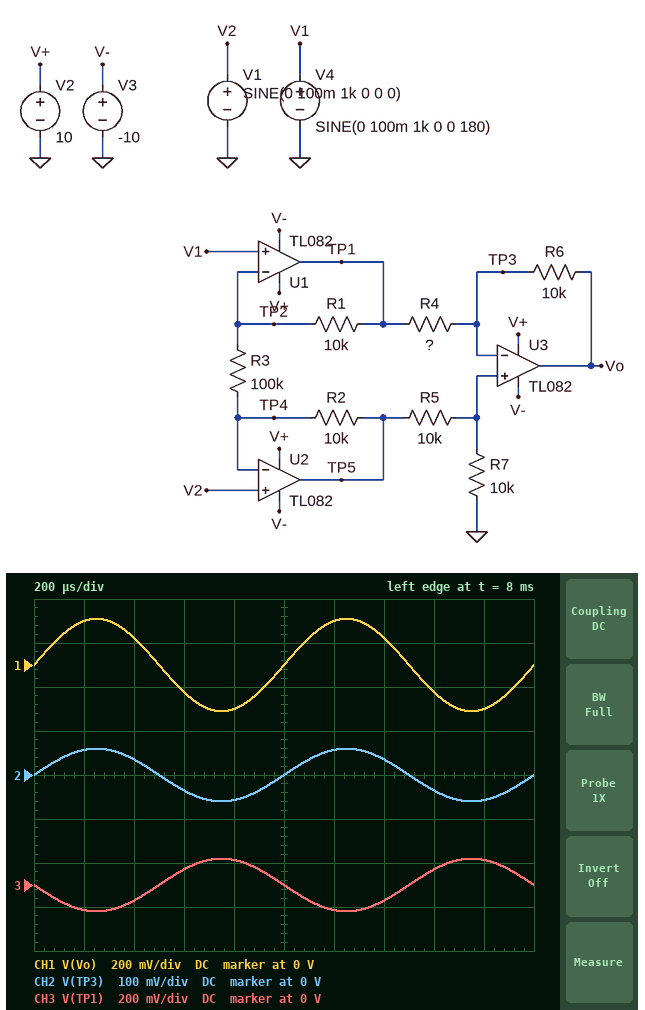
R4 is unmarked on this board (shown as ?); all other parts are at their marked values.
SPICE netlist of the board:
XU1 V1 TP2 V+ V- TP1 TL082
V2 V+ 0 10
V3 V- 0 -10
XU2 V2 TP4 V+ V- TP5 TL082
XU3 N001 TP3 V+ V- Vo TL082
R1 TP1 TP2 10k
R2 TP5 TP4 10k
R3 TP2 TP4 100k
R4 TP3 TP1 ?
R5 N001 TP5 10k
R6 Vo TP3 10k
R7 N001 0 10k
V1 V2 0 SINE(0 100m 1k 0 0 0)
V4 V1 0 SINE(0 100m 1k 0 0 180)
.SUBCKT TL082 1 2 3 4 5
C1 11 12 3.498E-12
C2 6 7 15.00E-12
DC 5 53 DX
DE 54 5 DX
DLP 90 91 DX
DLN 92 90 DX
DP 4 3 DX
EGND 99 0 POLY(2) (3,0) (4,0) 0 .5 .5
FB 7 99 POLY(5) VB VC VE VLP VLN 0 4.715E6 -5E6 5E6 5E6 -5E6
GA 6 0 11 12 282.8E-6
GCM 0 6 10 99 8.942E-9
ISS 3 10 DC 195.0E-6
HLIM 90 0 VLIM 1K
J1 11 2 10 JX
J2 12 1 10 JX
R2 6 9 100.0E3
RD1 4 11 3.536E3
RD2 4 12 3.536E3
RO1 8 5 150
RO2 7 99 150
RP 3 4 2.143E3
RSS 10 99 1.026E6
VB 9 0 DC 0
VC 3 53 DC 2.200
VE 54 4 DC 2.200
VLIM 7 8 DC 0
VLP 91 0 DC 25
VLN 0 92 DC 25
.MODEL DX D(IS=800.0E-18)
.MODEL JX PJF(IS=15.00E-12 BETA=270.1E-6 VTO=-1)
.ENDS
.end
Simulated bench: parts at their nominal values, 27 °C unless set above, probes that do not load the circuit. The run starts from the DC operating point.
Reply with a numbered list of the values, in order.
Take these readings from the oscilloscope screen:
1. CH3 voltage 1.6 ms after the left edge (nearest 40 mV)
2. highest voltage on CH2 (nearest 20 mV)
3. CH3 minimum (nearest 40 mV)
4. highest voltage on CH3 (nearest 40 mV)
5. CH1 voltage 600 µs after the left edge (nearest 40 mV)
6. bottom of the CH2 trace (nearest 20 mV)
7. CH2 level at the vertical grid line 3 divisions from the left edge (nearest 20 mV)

1. 80 mV
2. 60 mV
3. -120 mV
4. 120 mV
5. -120 mV
6. -60 mV
7. -40 mV
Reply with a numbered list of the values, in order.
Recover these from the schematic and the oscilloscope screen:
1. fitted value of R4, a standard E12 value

1. 12 kΩ
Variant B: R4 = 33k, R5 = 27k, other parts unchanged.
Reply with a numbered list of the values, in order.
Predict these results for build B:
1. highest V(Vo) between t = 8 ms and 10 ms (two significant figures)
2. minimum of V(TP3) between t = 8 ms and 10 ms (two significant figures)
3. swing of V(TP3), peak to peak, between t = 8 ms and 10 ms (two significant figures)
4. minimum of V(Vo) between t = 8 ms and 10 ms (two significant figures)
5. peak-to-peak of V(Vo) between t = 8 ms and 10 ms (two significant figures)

1. 79 mV
2. -32 mV
3. 65 mV
4. -79 mV
5. 160 mV
